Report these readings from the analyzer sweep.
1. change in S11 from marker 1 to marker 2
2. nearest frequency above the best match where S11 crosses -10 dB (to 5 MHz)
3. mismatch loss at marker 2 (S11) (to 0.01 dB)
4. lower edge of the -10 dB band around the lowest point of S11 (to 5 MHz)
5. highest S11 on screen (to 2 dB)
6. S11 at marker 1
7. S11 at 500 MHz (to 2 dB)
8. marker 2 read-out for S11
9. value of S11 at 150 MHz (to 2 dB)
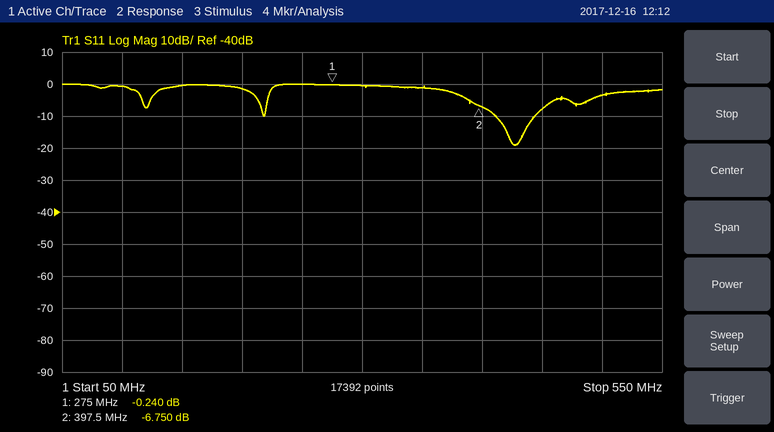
-6.510 dB
445 MHz
1.03 dB
410 MHz
0 dB
-0.240 dB
-4 dB
-6.750 dB
0 dB
